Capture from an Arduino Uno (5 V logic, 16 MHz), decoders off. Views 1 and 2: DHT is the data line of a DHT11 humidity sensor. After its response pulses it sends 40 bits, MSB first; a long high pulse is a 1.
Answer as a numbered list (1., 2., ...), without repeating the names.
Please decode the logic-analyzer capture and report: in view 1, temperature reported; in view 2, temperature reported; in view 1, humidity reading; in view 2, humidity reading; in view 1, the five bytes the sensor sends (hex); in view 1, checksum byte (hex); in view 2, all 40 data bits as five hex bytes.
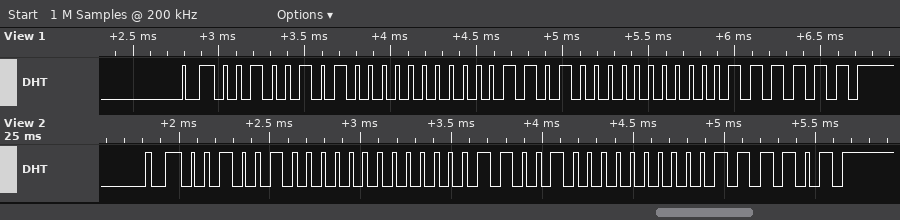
1. 26.0 °C
2. 25.0 °C
3. 37 %
4. 36 %
5. 25 00 1A 00 3F
6. 0x3F
7. 24 00 19 00 3D
